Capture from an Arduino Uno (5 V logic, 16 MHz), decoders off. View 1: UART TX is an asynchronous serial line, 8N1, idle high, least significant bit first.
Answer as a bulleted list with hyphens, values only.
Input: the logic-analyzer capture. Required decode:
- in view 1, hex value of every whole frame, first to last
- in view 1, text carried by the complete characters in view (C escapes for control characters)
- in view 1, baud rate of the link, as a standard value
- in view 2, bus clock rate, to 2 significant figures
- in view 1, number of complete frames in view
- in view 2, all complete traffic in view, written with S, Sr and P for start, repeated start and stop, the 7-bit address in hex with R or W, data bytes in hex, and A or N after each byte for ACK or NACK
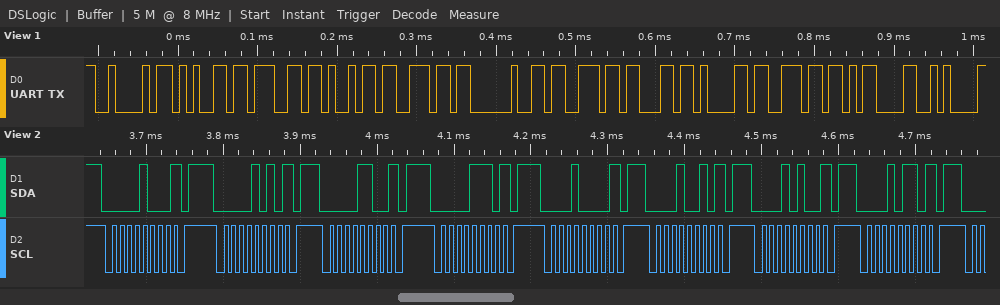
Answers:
- 42 65 67 69 6E 20 73 63 61 6E 0D 0A
- "Begin scan\r\n"
- 115200 baud
- 100 kHz
- 12
- S 04W N P S 05W N P S 06W N P S 07W N P S 08W N P S 09W N P S 0AW N P S 0BW N P
